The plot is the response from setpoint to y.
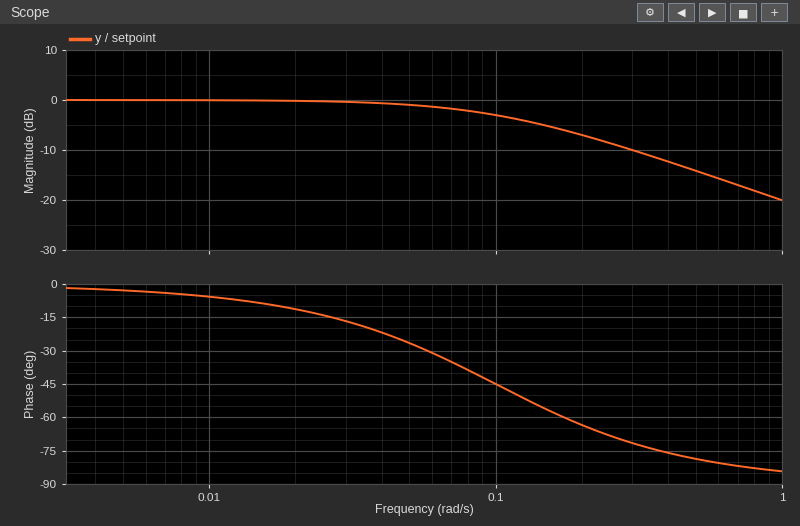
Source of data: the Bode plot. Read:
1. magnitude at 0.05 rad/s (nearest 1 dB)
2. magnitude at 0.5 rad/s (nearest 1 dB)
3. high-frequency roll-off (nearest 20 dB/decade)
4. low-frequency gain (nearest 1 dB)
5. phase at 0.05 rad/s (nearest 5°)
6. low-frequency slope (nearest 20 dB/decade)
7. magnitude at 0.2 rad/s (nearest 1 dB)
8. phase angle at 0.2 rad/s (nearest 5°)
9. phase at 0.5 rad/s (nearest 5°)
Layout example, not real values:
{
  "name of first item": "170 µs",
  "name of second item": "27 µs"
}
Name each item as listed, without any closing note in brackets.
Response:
{
  "magnitude at 0.05 rad/s": "-1 dB",
  "magnitude at 0.5 rad/s": "-14 dB",
  "high-frequency roll-off": "-20 dB/decade",
  "low-frequency gain": "0 dB",
  "phase at 0.05 rad/s": "-25°",
  "low-frequency slope": "0 dB/decade",
  "magnitude at 0.2 rad/s": "-7 dB",
  "phase angle at 0.2 rad/s": "-65°",
  "phase at 0.5 rad/s": "-80°"
}
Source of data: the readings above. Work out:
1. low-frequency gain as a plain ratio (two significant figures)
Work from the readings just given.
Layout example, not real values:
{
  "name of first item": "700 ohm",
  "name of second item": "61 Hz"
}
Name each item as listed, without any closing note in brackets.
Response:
{
  "low-frequency gain as a plain ratio": "1.0"
}
